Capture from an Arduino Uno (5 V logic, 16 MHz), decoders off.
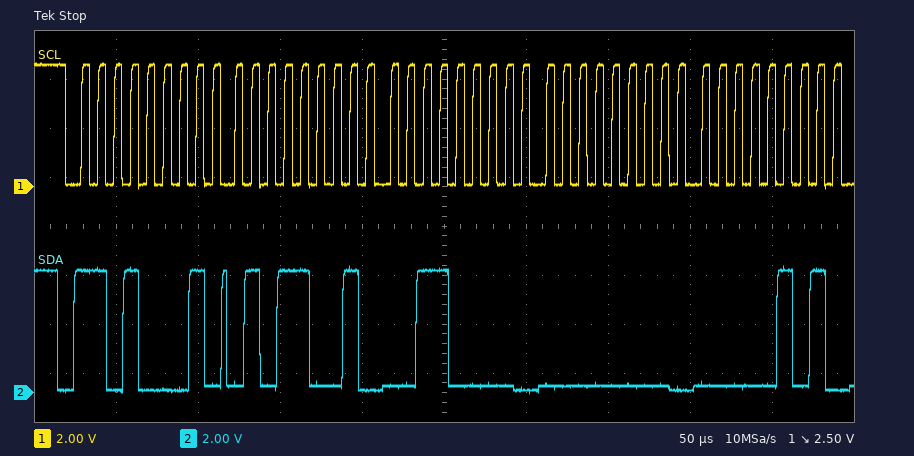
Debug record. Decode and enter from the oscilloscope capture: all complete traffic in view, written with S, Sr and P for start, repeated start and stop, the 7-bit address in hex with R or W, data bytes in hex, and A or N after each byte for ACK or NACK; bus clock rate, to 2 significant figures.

S 68R A 59 A 30 A 00 A 05 A
100 kHz
